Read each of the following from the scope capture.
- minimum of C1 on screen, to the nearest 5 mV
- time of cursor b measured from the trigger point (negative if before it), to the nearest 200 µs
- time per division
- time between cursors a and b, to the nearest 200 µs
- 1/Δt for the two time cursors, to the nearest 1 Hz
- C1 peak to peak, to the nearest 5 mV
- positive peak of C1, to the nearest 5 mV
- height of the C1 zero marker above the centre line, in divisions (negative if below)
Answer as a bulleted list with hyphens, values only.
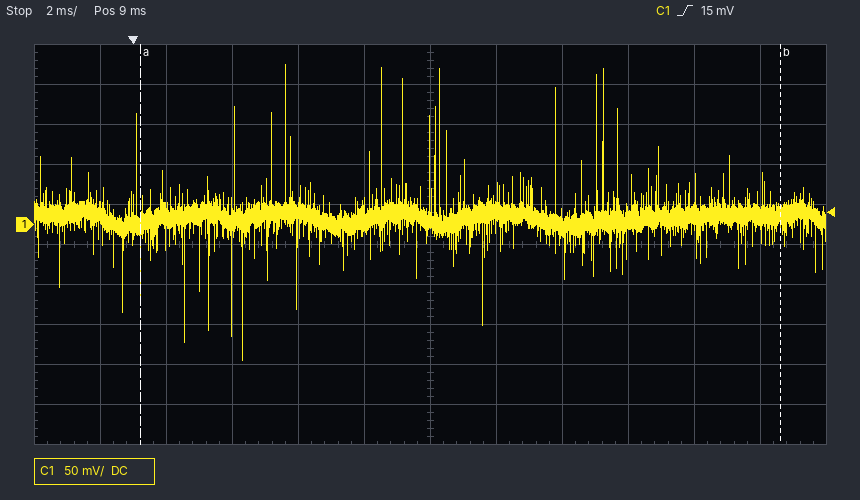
- -170 mV
- +19.6 ms
- 2 ms
- 19.4 ms
- 52 Hz
- 370 mV
- 200 mV
- +0.5 div
